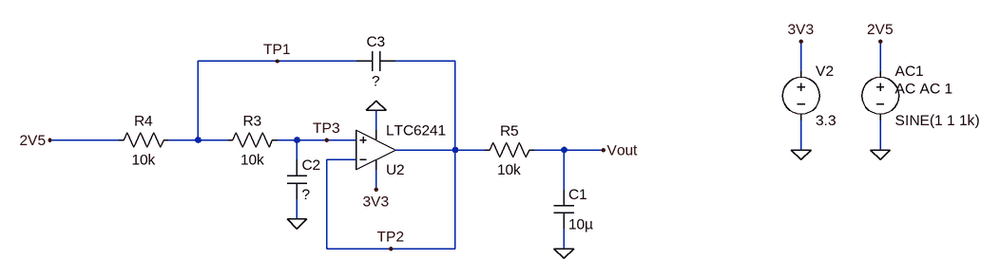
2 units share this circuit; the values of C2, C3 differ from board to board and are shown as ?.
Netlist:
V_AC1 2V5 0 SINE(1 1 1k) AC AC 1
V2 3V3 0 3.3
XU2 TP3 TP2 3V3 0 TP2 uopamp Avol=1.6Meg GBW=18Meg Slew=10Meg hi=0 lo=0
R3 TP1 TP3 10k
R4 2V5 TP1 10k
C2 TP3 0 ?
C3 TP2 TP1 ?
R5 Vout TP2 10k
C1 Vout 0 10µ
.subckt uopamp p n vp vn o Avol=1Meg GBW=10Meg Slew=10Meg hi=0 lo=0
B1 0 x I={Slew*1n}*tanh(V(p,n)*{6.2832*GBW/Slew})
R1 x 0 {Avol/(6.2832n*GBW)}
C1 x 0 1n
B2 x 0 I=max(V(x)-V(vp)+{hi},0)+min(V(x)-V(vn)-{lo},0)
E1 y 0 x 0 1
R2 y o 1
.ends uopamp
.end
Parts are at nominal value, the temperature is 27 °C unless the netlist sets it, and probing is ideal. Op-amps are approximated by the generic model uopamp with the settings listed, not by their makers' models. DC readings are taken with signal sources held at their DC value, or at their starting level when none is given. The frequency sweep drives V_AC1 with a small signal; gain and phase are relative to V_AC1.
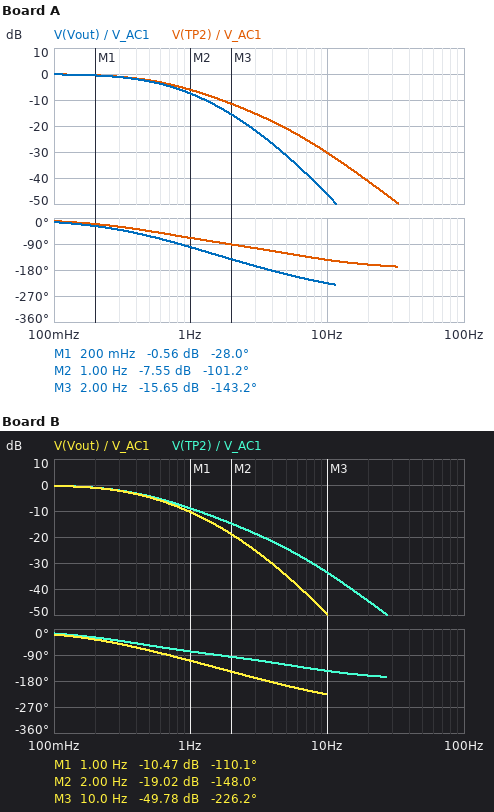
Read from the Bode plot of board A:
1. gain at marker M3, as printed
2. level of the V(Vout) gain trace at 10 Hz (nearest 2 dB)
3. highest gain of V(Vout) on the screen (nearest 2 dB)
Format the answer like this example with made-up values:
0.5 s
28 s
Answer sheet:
-15.65 dB
-46 dB
0 dB
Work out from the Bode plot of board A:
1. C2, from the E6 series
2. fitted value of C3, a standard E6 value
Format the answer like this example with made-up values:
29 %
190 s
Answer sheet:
15 µF
4.7 µF
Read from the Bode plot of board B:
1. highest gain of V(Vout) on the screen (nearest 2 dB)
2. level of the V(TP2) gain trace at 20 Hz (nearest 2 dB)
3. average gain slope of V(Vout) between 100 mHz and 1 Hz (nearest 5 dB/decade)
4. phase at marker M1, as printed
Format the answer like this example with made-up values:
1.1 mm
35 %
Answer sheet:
0 dB
-44 dB
-10 dB/decade
-110.1 deg
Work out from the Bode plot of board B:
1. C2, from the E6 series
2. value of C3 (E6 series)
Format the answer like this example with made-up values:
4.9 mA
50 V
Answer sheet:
22 µF
4.7 µF
